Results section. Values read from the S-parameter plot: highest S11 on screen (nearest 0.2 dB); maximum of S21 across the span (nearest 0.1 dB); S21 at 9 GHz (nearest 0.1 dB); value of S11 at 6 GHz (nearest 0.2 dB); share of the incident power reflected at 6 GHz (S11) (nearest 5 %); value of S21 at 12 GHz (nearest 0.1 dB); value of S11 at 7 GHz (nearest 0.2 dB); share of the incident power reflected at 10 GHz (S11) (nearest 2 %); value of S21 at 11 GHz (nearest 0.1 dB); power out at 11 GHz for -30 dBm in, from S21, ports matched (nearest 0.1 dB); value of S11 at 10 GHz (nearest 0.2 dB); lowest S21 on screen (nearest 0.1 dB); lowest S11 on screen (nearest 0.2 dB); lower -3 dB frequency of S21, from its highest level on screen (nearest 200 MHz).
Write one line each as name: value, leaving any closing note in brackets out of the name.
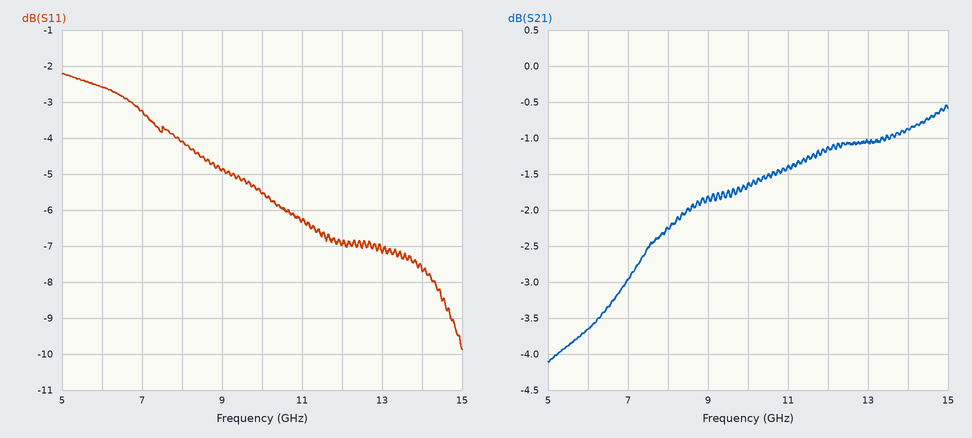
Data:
highest S11 on screen: -2.2 dB
maximum of S21 across the span: -0.5 dB
S21 at 9 GHz: -1.8 dB
value of S11 at 6 GHz: -2.6 dB
share of the incident power reflected at 6 GHz (S11): 55 %
value of S21 at 12 GHz: -1.1 dB
value of S11 at 7 GHz: -3.2 dB
share of the incident power reflected at 10 GHz (S11): 28 %
value of S21 at 11 GHz: -1.4 dB
power out at 11 GHz for -30 dBm in, from S21, ports matched: -31.4 dBm
value of S11 at 10 GHz: -5.6 dB
lowest S21 on screen: -4.1 dB
lowest S11 on screen: -9.8 dB
lower -3 dB frequency of S21, from its highest level on screen: 6.2 GHz
